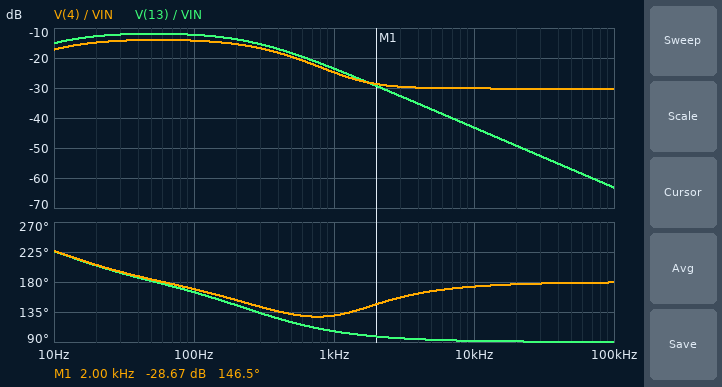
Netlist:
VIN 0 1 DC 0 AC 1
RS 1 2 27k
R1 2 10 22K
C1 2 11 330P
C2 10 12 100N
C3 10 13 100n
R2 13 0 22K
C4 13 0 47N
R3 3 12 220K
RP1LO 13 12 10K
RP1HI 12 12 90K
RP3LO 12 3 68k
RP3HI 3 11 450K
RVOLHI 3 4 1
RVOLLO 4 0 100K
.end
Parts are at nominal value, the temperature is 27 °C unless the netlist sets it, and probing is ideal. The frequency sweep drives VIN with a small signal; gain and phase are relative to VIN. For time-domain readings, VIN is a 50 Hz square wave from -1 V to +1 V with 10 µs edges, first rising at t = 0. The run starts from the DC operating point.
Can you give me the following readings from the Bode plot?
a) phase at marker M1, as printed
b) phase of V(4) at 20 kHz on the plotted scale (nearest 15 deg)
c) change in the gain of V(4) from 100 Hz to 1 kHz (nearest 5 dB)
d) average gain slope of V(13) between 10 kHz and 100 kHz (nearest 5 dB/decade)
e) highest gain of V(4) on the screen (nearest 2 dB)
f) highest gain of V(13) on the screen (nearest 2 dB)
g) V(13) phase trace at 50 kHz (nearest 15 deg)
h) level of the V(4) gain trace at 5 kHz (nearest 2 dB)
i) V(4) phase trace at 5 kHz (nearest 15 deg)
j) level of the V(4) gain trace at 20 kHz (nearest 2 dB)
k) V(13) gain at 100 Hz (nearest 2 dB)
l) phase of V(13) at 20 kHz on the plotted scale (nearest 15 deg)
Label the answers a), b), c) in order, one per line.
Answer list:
a) 146.5 deg
b) 180 deg
c) -10 dB
d) -20 dB/decade
e) -14 dB
f) -12 dB
g) 90 deg
h) -30 dB
i) 165 deg
j) -30 dB
k) -12 dB
l) 90 deg
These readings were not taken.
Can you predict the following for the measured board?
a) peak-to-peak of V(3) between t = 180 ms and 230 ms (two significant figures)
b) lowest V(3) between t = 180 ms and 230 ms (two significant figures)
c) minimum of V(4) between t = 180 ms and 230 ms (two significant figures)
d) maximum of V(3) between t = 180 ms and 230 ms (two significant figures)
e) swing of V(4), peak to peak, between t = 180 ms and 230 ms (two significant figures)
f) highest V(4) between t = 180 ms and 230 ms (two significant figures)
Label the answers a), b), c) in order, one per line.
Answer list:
a) 480 mV
b) -240 mV
c) -240 mV
d) 240 mV
e) 480 mV
f) 240 mV
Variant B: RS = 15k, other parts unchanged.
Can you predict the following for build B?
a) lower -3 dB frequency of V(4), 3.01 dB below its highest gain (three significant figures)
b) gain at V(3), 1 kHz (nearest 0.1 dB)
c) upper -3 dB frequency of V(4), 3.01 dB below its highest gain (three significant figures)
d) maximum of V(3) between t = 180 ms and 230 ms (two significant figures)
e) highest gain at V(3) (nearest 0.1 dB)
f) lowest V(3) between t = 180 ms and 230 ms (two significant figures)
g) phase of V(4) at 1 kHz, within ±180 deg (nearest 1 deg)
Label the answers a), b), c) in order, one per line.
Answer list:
a) 12.4 Hz
b) -22.4 dB
c) 348 Hz
d) 300 mV
e) -12.4 dB
f) -300 mV
g) 132 deg
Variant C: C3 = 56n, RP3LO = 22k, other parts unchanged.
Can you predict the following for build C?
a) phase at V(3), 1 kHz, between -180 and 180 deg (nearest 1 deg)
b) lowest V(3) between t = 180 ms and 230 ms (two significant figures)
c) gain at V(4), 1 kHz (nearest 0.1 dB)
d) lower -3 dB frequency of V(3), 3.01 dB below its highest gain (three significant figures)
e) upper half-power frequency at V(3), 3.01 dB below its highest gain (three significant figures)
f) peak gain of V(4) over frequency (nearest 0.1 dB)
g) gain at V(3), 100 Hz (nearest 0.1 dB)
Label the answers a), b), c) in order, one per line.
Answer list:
a) 122 deg
b) -310 mV
c) -20.7 dB
d) 13.1 Hz
e) 369 Hz
f) -12.0 dB
g) -12.2 dB
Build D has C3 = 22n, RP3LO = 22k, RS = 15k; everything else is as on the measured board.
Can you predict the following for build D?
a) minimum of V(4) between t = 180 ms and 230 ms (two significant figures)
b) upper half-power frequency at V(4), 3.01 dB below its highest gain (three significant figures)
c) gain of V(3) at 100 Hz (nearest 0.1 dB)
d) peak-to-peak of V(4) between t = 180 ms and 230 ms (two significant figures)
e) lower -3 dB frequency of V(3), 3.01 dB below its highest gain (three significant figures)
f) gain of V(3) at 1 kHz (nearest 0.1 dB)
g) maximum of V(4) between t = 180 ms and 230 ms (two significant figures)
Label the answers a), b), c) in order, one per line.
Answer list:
a) -410 mV
b) 508 Hz
c) -10.4 dB
d) 820 mV
e) 18.7 Hz
f) -15.7 dB
g) 410 mV
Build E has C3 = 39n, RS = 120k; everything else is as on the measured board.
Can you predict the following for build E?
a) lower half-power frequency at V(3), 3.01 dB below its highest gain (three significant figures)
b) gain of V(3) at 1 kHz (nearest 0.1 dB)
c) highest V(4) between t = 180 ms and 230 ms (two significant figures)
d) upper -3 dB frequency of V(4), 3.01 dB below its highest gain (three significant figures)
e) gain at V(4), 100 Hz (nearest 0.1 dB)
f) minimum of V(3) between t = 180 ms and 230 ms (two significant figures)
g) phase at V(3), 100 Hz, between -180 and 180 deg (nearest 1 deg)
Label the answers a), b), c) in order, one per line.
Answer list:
a) 6.52 Hz
b) -30.7 dB
c) 100 mV
d) 262 Hz
e) -21.1 dB
f) -100 mV
g) 165 deg
